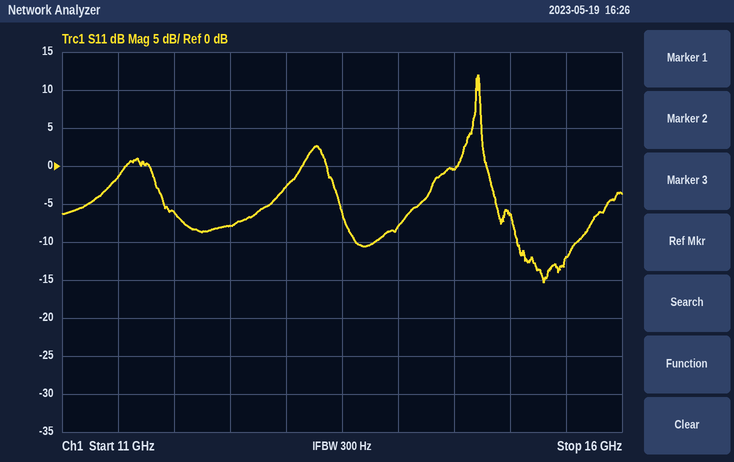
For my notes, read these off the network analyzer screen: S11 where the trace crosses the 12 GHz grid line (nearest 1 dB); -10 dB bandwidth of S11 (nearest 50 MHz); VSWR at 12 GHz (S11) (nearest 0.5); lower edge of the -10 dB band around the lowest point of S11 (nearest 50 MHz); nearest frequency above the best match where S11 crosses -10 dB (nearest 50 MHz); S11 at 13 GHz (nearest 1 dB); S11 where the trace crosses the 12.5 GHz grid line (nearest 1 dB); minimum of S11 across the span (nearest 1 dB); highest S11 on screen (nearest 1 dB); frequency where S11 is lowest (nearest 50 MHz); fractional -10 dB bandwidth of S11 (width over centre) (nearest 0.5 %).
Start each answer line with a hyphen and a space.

- -6 dB
- 550 MHz
- 3.0
- 15.05 GHz
- 15.60 GHz
- -3 dB
- -8 dB
- -15 dB
- 12 dB
- 15.30 GHz
- 3.5 %
